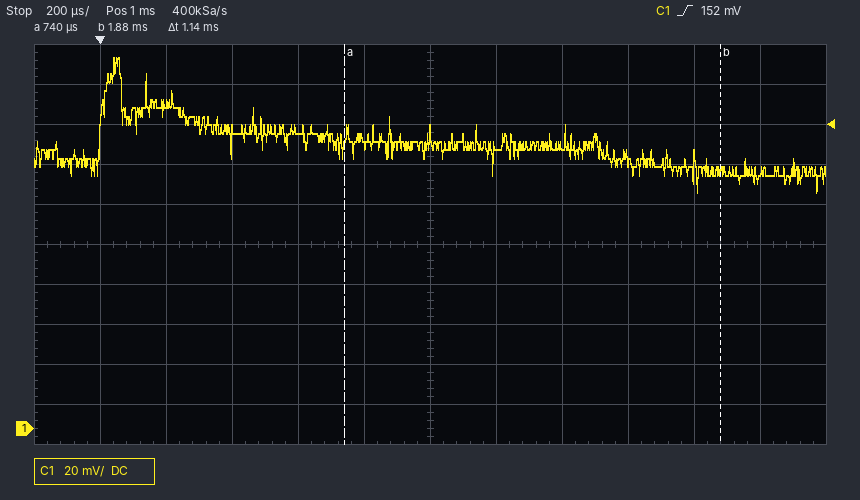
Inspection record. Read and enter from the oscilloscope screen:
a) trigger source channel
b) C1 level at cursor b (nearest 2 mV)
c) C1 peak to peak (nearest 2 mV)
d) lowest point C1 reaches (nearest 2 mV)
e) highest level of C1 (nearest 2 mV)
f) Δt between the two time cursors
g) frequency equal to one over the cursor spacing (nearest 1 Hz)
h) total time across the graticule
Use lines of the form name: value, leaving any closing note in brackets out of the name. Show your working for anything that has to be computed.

trigger source channel: C1
C1 level at cursor b: 128 mV
C1 peak to peak: 186 mV − (118 mV) = 68 mV
lowest point C1 reaches: 118 mV
highest level of C1: 186 mV
Δt between the two time cursors: 1.14 ms
frequency equal to one over the cursor spacing: 1 / 1.14 ms ≈ 877 Hz
total time across the graticule: 2.4 ms
